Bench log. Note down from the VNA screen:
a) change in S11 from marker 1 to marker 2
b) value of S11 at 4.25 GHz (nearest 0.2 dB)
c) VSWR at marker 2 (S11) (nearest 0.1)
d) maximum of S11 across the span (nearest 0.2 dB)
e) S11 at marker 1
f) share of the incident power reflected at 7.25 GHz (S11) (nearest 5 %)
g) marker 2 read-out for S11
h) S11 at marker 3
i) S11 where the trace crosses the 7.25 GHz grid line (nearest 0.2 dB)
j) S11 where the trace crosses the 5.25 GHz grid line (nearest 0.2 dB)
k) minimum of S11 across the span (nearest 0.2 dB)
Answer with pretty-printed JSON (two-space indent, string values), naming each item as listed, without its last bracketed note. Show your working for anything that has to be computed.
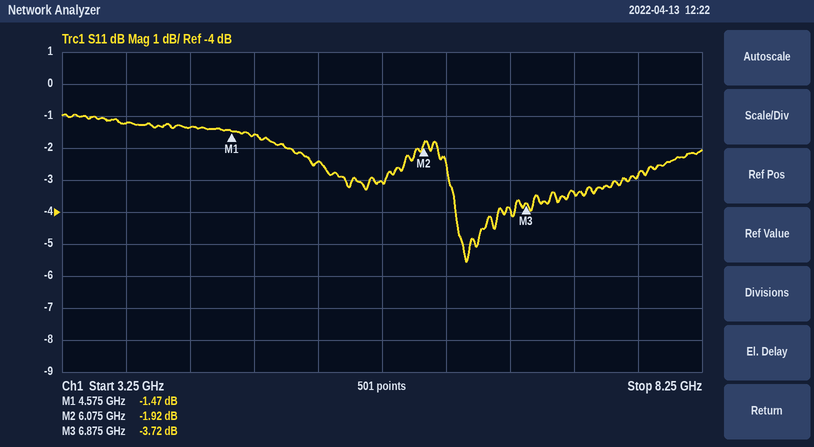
{
  "change in S11 from marker 1 to marker 2": "-1.92 − (-1.47) = -0.45 dB",
  "value of S11 at 4.25 GHz": "-1.4 dB",
  "VSWR at marker 2 (S11)": "(1 + 0.8017)/(1 − 0.8017) ≈ 9.1",
  "maximum of S11 across the span": "-1.0 dB",
  "S11 at marker 1": "-1.47 dB",
  "share of the incident power reflected at 7.25 GHz (S11)": "10^(-3.4/10) ≈ 45.7 %, so 45 % to the nearest 5 %",
  "marker 2 read-out for S11": "-1.92 dB",
  "S11 at marker 3": "-3.72 dB",
  "S11 where the trace crosses the 7.25 GHz grid line": "-3.4 dB",
  "S11 where the trace crosses the 5.25 GHz grid line": "-2.4 dB",
  "minimum of S11 across the span": "-5.6 dB"
}
